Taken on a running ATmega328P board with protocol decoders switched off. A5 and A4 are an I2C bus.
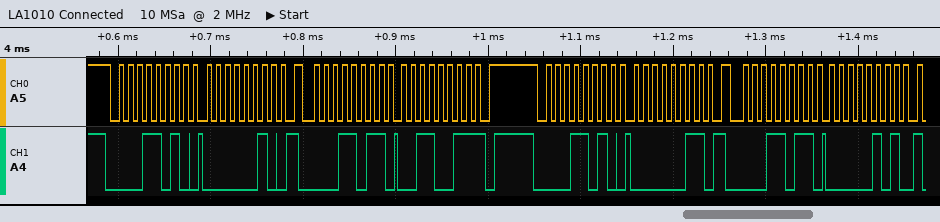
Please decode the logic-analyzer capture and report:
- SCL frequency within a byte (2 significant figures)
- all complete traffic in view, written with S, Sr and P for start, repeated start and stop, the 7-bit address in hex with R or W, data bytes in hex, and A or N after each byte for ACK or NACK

100 kHz
S 0DW A 02 A Sr 0DR A 33 N P S 0DW A 03 A Sr 0DR A 05 A
